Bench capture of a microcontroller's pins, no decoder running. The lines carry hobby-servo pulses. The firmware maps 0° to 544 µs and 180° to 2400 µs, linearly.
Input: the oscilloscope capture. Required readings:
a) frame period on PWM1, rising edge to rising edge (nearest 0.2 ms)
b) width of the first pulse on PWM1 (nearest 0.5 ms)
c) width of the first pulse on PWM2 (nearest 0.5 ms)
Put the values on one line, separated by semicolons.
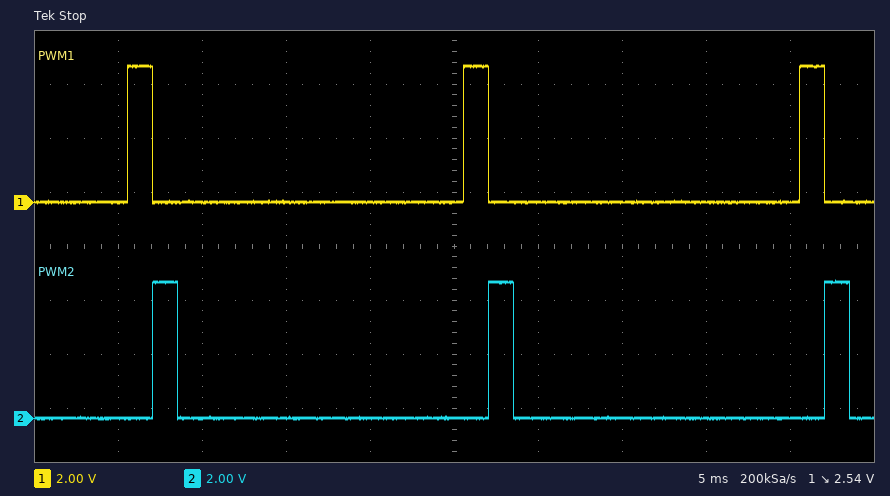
20.0 ms; 1.5 ms; 1.5 ms
